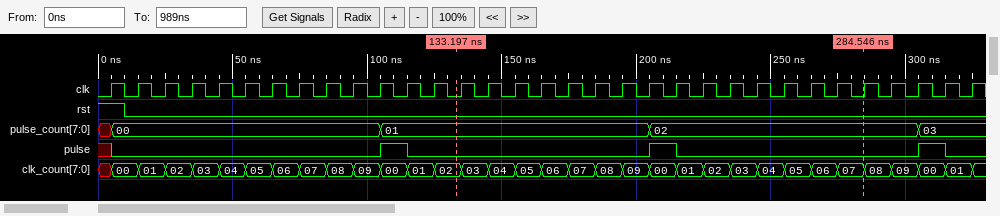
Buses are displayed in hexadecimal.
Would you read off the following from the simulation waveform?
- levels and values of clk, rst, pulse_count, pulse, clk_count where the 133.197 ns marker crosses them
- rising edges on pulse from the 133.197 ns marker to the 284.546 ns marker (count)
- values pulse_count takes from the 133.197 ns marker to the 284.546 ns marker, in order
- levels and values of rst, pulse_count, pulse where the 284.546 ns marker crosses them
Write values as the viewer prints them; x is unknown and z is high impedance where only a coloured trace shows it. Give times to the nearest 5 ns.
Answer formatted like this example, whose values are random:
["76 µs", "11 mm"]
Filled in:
["clk=0, rst=0, pulse_count=01, pulse=0, clk_count=02", "1", "01, 02", "rst=0, pulse_count=02, pulse=0"]
